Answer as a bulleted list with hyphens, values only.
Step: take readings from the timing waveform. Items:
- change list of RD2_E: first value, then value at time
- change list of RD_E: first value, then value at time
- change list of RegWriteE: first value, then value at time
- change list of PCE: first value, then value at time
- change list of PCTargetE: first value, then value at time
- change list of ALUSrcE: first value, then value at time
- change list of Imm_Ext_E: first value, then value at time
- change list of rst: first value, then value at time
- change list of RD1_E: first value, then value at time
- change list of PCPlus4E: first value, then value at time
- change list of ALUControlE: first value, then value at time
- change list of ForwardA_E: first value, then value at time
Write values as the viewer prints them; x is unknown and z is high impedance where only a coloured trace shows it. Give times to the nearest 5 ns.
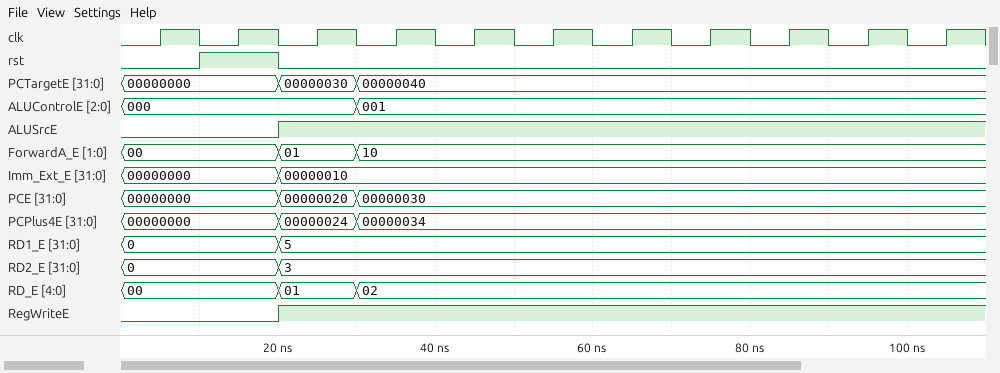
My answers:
- 0, 3 at 20 ns
- 00, 01 at 20 ns, 02 at 30 ns
- 0, 1 at 20 ns
- 00000000, 00000020 at 20 ns, 00000030 at 30 ns
- 00000000, 00000030 at 20 ns, 00000040 at 30 ns
- 0, 1 at 20 ns
- 00000000, 00000010 at 20 ns
- 0, 1 at 10 ns, 0 at 20 ns
- 0, 5 at 20 ns
- 00000000, 00000024 at 20 ns, 00000034 at 30 ns
- 000, 001 at 30 ns
- 00, 01 at 20 ns, 10 at 30 ns
